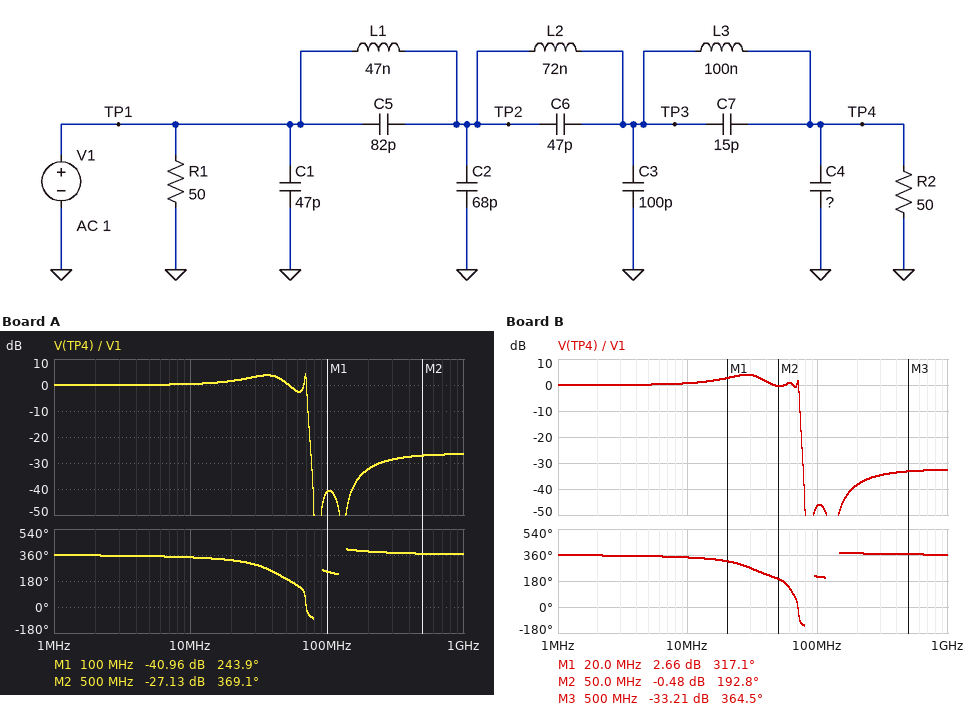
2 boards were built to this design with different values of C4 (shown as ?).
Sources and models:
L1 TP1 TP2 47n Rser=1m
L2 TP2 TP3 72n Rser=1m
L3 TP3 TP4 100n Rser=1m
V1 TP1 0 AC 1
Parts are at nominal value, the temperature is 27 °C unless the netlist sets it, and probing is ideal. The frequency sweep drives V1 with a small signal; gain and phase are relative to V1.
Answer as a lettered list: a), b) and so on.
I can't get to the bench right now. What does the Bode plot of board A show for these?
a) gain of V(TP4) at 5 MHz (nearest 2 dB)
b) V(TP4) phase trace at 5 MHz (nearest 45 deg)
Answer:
a) 0 dB
b) 360 deg
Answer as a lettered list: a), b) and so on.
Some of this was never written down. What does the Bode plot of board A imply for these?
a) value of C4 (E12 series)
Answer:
a) 27 pF
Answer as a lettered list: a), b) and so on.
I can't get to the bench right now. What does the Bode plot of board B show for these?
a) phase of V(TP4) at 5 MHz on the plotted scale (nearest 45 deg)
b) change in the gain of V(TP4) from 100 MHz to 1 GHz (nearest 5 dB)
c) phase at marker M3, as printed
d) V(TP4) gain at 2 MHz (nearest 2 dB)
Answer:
a) 360 deg
b) 15 dB
c) 364.5 deg
d) 0 dB
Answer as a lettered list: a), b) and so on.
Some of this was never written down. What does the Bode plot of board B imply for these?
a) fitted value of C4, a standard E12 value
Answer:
a) 68 pF
